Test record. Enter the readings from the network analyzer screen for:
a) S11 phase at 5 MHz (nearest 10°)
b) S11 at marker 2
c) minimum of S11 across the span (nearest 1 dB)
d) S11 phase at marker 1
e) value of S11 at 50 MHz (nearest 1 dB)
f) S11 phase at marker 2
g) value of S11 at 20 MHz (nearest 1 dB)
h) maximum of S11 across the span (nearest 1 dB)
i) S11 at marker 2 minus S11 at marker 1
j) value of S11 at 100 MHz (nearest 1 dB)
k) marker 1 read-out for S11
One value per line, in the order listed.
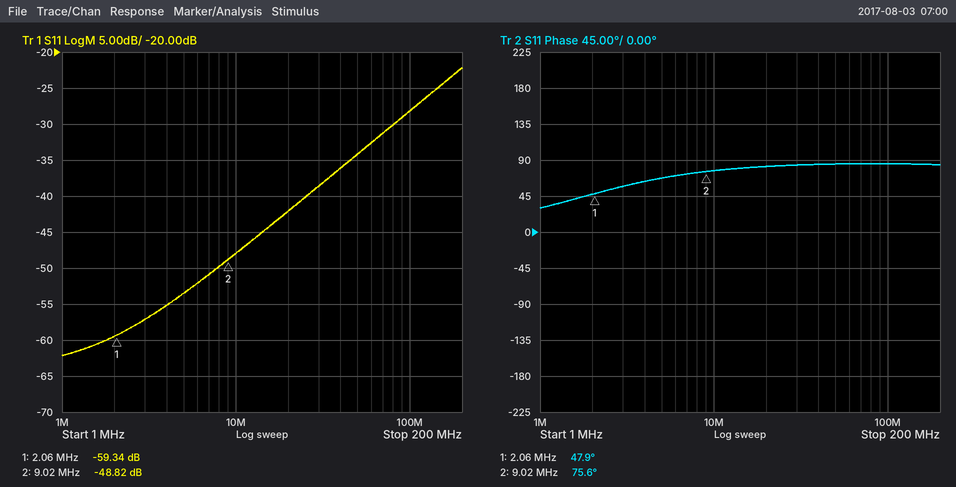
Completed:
70°
-48.82 dB
-62 dB
47.9°
-34 dB
75.6°
-42 dB
-22 dB
10.52 dB
-28 dB
-59.34 dB
